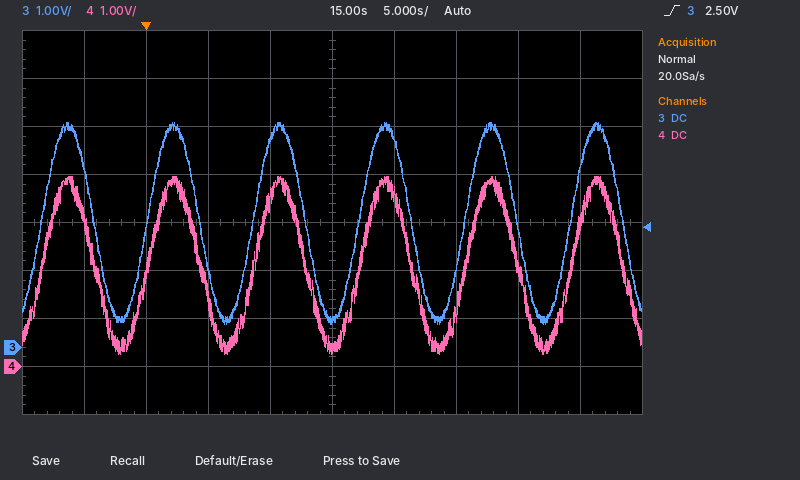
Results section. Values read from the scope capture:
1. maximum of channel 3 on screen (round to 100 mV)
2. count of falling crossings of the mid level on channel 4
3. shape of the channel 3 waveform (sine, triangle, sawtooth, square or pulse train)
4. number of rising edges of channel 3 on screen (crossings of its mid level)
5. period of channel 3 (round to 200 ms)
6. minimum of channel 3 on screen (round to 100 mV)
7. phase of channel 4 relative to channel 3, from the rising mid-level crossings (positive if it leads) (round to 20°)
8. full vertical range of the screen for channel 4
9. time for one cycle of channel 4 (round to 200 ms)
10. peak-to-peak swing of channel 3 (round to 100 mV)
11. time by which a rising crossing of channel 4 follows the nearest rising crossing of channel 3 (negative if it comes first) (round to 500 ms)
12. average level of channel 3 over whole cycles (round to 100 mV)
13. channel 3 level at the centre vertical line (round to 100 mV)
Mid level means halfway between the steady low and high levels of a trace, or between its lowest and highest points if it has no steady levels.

4.7 V
6
sine
6
8.6 s
500 mV
0°
8 V
8.6 s
4.2 V
0.0 s
2.6 V
600 mV
